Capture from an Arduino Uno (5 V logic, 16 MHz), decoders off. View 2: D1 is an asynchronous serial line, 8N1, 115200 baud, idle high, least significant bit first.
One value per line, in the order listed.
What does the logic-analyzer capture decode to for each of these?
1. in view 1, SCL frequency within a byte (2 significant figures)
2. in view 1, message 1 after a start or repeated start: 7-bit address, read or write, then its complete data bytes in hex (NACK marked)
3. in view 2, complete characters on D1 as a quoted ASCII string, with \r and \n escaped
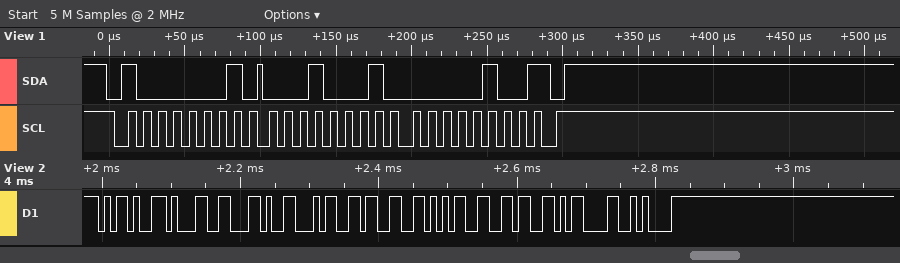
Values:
100 kHz
0x40 read: 11 04 NACK
"-1,4356\r\n"
